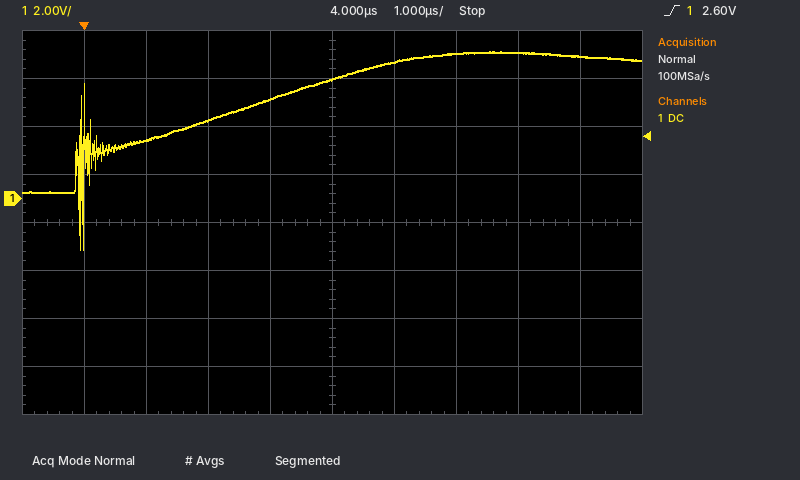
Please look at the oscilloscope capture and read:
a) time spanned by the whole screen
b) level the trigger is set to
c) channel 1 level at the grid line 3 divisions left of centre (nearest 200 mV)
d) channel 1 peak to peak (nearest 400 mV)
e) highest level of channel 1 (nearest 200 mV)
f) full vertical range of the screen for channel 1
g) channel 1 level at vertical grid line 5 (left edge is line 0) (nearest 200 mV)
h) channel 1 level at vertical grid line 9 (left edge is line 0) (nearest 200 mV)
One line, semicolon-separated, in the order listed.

10 µs; 2.60 V; 2.4 V; 8.4 V; 6.2 V; 16 V; 5.0 V; 6.0 V
